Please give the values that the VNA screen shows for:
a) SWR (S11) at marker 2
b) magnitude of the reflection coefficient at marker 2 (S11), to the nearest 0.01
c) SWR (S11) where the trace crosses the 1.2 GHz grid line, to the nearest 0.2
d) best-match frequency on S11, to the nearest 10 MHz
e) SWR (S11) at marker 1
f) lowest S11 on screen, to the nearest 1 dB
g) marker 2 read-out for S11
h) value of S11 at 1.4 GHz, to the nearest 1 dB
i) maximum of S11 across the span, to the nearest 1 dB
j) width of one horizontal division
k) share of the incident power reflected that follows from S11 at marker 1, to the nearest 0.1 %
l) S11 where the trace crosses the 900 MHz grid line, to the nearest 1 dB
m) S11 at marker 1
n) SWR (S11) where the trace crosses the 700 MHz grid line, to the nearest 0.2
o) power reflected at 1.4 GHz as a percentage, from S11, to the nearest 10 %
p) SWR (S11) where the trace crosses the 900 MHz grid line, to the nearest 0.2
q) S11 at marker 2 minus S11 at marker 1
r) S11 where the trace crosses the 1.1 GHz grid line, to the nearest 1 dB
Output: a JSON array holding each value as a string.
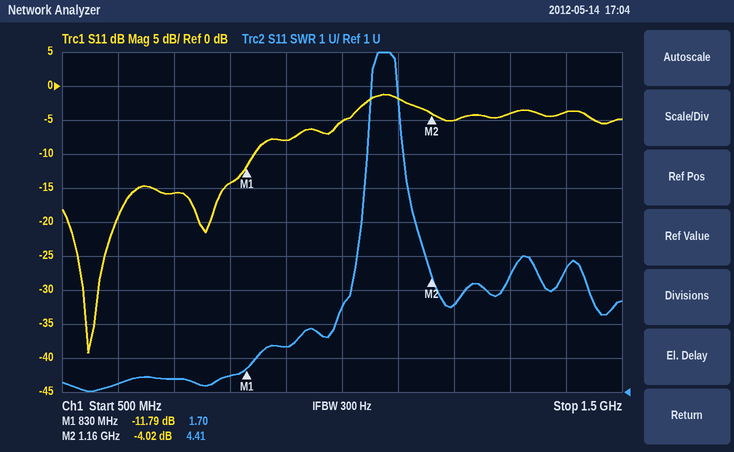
["4.41", "0.63", "3.6", "550 MHz", "1.70", "-39 dB", "-4.02 dB", "-4 dB", "-1 dB", "100 MHz", "6.6 %", "-8 dB", "-11.79 dB", "1.4", "40 %", "2.4", "7.77 dB", "-2 dB"]
